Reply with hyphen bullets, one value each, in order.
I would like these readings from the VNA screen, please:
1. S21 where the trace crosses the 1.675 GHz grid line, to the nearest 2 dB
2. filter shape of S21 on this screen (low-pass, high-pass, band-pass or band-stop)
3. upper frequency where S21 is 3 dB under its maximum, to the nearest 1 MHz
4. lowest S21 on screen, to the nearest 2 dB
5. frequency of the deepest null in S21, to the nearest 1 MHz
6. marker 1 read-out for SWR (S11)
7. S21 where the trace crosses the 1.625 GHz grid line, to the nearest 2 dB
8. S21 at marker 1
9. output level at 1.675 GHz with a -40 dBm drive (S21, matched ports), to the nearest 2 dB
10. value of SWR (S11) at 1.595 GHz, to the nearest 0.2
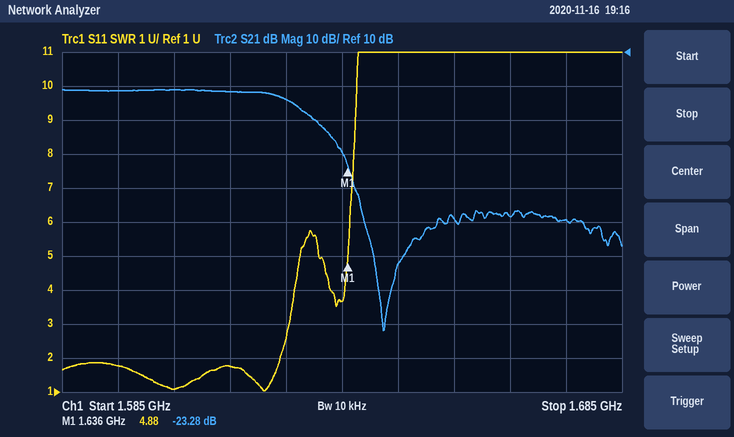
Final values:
- -40 dB
- low-pass
- 1.625 GHz
- -72 dB
- 1.642 GHz
- 4.88
- -4 dB
- -23.28 dB
- -80 dBm
- 1.8
